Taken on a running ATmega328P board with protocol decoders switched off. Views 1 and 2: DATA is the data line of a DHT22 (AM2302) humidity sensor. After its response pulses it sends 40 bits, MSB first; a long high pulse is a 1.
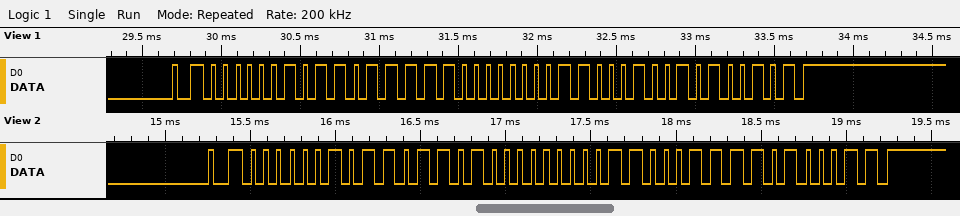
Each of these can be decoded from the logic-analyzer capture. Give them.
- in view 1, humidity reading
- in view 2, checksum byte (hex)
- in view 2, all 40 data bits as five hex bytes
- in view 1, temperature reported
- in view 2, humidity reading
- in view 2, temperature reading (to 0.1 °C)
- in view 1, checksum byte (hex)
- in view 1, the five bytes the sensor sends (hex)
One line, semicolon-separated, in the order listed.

73.5 %; 0xA3; 02 DA 00 C7 A3; 19.6 °C; 73.0 %; 19.9 °C; 0xA5; 02 DF 00 C4 A5
